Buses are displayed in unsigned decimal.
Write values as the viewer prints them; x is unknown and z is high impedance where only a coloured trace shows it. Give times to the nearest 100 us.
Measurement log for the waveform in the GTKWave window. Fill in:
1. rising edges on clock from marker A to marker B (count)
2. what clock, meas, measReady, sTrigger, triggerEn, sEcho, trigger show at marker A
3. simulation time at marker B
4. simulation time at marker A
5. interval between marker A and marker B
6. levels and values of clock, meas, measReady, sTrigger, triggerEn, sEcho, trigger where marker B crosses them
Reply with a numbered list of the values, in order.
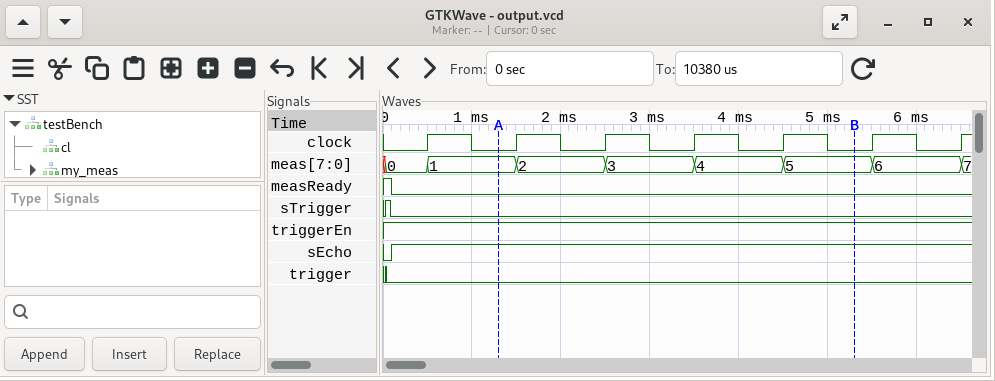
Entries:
1. 4
2. clock=0, meas=1, measReady=0, sTrigger=0, triggerEn=1, sEcho=1, trigger=0
3. 5300 us
4. 1300 us
5. 4000 us
6. clock=0, meas=5, measReady=0, sTrigger=0, triggerEn=1, sEcho=1, trigger=0
